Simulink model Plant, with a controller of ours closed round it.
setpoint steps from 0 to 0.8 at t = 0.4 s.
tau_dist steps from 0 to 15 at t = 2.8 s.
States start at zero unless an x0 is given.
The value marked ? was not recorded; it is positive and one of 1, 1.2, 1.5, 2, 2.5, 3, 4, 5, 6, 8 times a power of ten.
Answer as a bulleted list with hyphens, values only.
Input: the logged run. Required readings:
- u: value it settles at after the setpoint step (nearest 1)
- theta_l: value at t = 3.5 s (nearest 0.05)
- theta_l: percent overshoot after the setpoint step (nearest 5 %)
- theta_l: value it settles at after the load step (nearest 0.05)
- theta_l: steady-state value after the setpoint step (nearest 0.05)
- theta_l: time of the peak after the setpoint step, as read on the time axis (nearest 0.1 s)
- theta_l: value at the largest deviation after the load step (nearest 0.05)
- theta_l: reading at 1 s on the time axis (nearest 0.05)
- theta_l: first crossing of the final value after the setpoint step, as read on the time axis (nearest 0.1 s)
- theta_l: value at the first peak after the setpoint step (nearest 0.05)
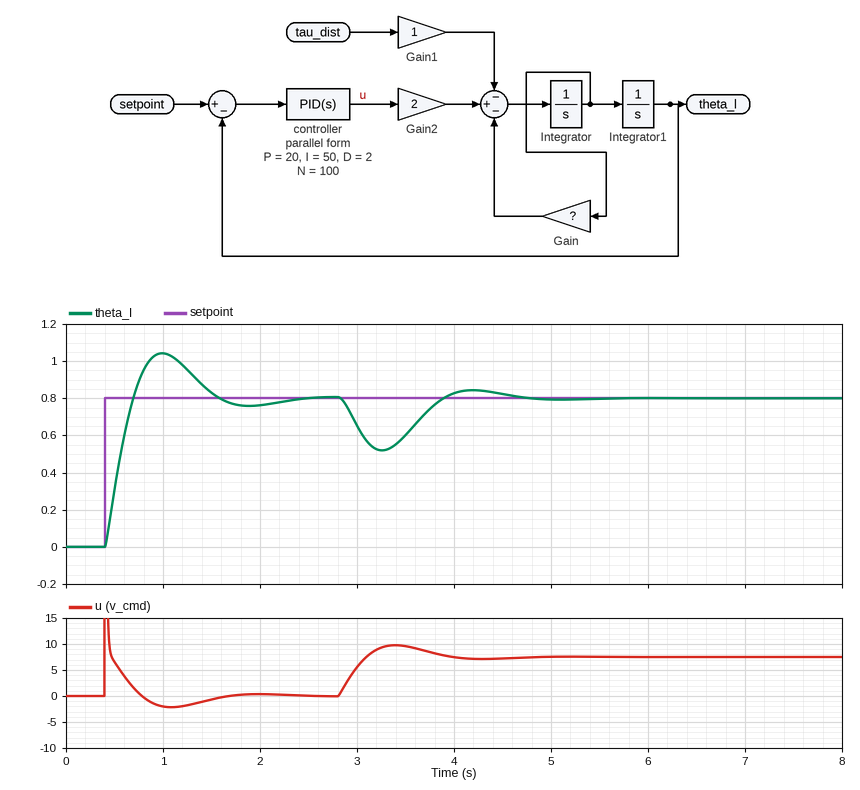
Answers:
- 0
- 0.60
- 30 %
- 0.80
- 0.80
- 1.0 s
- 0.50
- 1.05
- 0.7 s
- 1.05
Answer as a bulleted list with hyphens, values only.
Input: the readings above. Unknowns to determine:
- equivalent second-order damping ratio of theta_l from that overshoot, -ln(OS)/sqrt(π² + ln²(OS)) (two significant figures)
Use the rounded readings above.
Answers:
- 0.36
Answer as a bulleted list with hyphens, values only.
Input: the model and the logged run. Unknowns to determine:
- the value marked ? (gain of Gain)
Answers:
- 6
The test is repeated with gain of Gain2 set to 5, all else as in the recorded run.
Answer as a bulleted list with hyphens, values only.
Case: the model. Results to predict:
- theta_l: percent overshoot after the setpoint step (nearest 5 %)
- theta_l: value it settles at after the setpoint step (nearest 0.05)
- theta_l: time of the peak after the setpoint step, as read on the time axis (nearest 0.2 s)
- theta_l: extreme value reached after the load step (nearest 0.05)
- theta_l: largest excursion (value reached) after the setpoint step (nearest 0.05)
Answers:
- 20 %
- 0.80
- 0.8 s
- 0.70
- 0.95
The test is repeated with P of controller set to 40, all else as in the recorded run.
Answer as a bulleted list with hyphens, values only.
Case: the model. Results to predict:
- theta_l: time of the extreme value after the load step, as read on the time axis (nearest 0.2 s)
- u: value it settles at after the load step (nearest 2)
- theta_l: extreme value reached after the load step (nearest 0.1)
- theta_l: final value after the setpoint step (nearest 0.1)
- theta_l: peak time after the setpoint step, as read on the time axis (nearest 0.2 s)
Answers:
- 3.2 s
- 8
- 0.6
- 0.8
- 0.8 s
